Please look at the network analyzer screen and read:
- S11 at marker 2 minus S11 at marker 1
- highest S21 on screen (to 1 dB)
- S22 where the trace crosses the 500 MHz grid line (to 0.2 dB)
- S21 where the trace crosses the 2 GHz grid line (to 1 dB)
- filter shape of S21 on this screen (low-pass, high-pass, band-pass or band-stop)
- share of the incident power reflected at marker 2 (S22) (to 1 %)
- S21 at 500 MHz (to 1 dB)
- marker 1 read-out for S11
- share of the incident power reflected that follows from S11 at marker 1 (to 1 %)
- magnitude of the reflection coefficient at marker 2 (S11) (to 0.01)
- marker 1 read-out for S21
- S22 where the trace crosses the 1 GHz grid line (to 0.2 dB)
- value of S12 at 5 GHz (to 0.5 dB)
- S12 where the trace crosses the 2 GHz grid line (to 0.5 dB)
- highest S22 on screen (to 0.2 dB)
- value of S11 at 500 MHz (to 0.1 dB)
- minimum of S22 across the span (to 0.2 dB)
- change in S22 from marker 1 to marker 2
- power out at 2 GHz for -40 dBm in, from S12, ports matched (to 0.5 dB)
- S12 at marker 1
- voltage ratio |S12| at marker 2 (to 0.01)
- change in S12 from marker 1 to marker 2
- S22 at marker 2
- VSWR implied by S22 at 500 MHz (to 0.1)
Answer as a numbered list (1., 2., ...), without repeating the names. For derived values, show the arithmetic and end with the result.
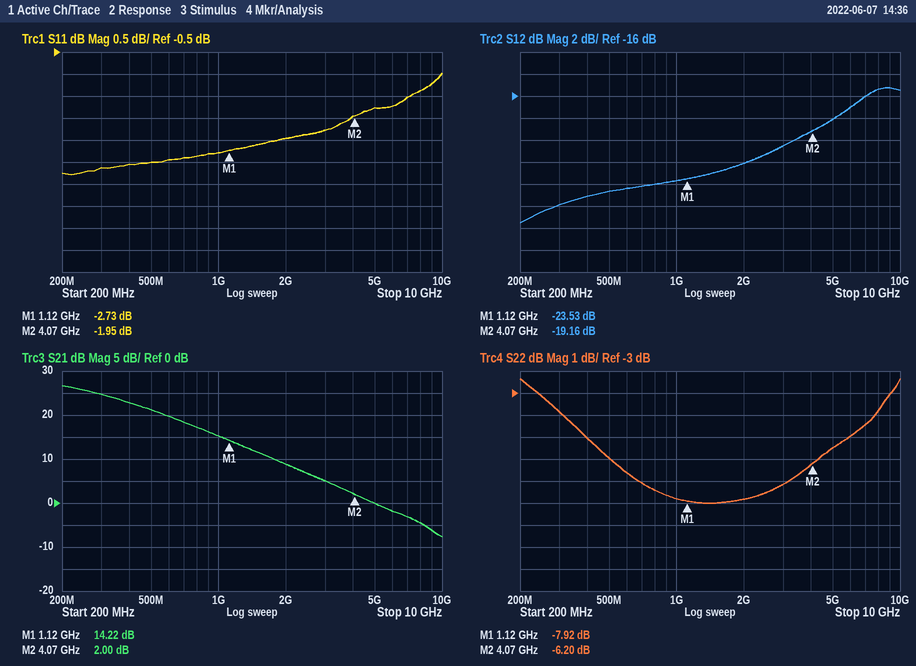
1. -1.95 − (-2.73) = 0.78 dB
2. 27 dB
3. -6.0 dB
4. 9 dB
5. low-pass
6. 10^(-6.2/10) ≈ 24 %
7. 21 dB
8. -2.73 dB
9. 10^(-2.73/10) ≈ 53 %
10. 10^(-1.95/20) ≈ 0.80
11. 14.22 dB
12. -7.8 dB
13. -18.0 dB
14. -22.0 dB
15. -2.4 dB
16. -3.0 dB
17. -8.0 dB
18. -6.2 − (-7.92) = 1.72 dB
19. -40 dBm + (-22.0 dB) = -62.0 dBm
20. -23.53 dB
21. 10^(-19.16/20) ≈ 0.11
22. -19.16 − (-23.53) = 4.37 dB
23. -6.20 dB
24. |Γ| = 10^(-6/20) = 0.5012; VSWR = (1 + 0.5012)/(1 − 0.5012) ≈ 3.0
